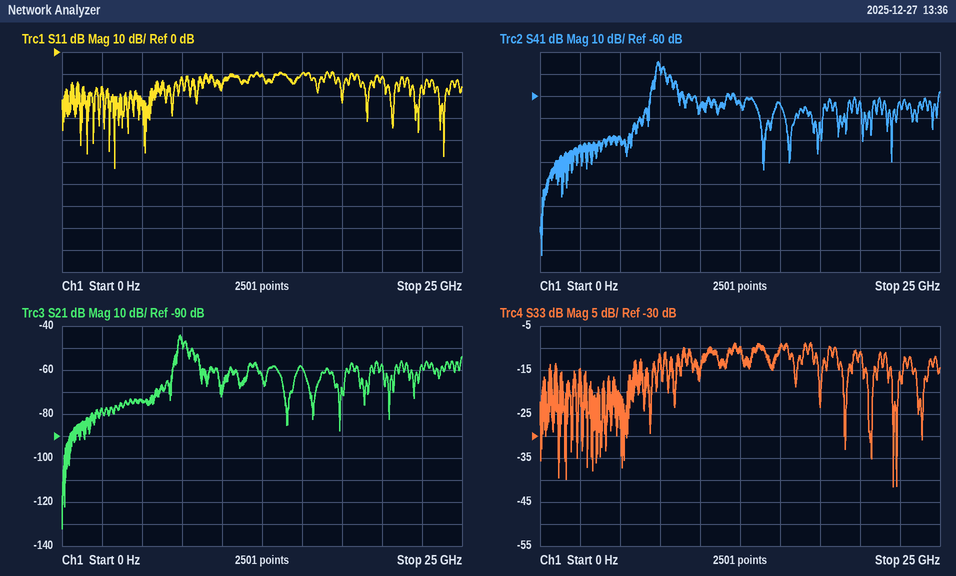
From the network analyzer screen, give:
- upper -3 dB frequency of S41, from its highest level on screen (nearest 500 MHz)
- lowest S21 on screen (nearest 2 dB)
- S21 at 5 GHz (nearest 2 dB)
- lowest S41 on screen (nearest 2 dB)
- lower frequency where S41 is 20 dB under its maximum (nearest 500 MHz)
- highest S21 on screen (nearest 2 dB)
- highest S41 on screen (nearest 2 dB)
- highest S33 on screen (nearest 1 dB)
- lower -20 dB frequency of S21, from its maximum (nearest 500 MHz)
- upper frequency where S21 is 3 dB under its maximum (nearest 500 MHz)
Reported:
7.5 GHz
-132 dB
-74 dB
-132 dB
7.0 GHz
-44 dB
-44 dB
-9 dB
7.0 GHz
7.5 GHz
